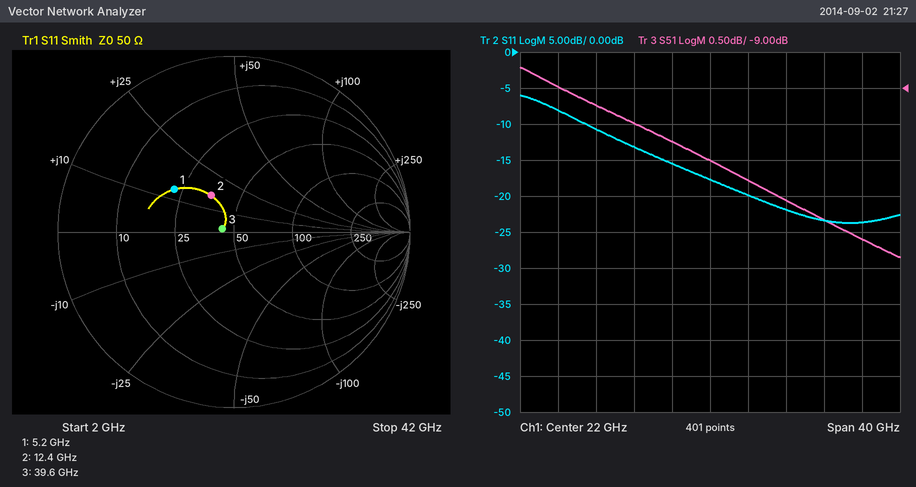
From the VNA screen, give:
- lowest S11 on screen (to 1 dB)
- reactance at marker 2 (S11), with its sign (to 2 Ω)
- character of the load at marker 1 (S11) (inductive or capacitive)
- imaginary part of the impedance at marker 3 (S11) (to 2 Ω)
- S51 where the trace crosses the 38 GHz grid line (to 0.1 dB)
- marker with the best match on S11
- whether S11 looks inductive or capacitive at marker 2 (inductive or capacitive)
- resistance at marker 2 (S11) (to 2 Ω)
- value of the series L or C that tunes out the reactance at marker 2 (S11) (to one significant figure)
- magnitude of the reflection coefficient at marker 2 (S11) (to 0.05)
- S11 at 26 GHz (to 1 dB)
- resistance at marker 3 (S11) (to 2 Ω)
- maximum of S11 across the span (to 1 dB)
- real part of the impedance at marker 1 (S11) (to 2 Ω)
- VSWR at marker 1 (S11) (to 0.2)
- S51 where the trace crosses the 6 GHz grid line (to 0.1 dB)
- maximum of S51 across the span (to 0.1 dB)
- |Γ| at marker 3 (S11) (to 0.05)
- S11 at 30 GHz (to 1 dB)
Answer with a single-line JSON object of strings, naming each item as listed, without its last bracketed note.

{"lowest S11 on screen": "-24 dB", "reactance at marker 2 (S11), with its sign": "+16 Ω", "character of the load at marker 1 (S11)": "inductive", "imaginary part of the impedance at marker 3 (S11)": "+2 Ω", "S51 where the trace crosses the 38 GHz grid line": "-11.1 dB", "marker with the best match on S11": "marker 3", "whether S11 looks inductive or capacitive at marker 2": "inductive", "resistance at marker 2 (S11)": "36 Ω", "value of the series L or C that tunes out the reactance at marker 2 (S11)": "800 fF", "magnitude of the reflection coefficient at marker 2 (S11)": "0.25", "S11 at 26 GHz": "-20 dB", "resistance at marker 3 (S11)": "44 Ω", "maximum of S11 across the span": "-6 dB", "real part of the impedance at marker 1 (S11)": "22 Ω", "VSWR at marker 1 (S11)": "2.4", "S51 where the trace crosses the 6 GHz grid line": "-9.0 dB", "maximum of S51 across the span": "-8.7 dB", "|Γ| at marker 3 (S11)": "0.05", "S11 at 30 GHz": "-22 dB"}
